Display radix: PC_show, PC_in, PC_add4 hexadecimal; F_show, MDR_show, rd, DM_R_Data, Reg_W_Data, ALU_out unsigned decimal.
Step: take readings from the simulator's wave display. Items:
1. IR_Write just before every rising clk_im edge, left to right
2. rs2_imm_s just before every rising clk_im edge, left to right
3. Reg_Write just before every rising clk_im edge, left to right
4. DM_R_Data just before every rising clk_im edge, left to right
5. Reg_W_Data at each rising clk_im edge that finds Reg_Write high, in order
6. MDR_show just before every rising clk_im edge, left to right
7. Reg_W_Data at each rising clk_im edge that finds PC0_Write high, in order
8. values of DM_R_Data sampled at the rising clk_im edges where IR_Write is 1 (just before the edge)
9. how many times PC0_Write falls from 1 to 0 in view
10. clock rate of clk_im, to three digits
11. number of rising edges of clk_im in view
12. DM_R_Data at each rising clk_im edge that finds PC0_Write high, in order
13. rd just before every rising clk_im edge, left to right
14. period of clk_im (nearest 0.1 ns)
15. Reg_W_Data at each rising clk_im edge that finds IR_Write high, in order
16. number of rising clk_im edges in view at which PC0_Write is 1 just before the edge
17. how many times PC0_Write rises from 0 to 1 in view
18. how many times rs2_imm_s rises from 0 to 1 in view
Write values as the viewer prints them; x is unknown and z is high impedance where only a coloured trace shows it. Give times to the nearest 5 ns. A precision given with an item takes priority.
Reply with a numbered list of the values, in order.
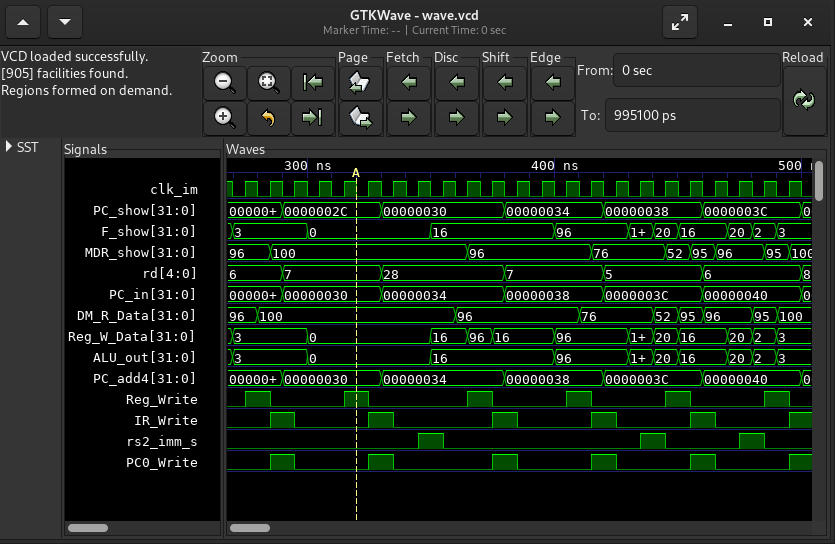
1. 0 0 1 0 0 0 1 0 0 0 0 1 0 0 0 1 0 0 0 1 0 0 0
2. 0 0 0 0 0 0 0 0 1 0 0 0 0 0 0 0 0 1 0 0 0 1 0
3. 0 1 0 0 0 1 0 0 0 0 1 0 0 0 1 0 0 0 1 0 0 0 1
4. 96, 100, 100, 100, 100, 100, 100, 100, 100, 96, 96, 96, 96, 96, 76, 76, 76, 52, 95, 96, 96, 95, 100
5. 3, 0, 96, 96, 16, 3
6. 96, 96, 100, 100, 100, 100, 100, 100, 100, 100, 96, 96, 96, 96, 96, 76, 76, 76, 52, 95, 96, 96, 95
7. 3, 0, 16, 96, 16
8. 100, 100, 96, 76, 96
9. 5
10. 100 MHz
11. 23
12. 100, 100, 96, 76, 96
13. 6, 6, 7, 7, 7, 7, 28, 28, 28, 28, 28, 7, 7, 7, 7, 5, 5, 5, 5, 6, 6, 6, 6
14. 10 ns
15. 3, 0, 16, 96, 16
16. 5
17. 6
18. 3
